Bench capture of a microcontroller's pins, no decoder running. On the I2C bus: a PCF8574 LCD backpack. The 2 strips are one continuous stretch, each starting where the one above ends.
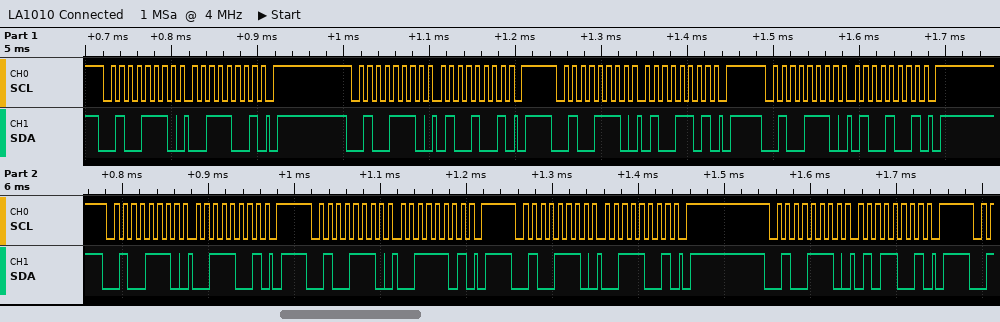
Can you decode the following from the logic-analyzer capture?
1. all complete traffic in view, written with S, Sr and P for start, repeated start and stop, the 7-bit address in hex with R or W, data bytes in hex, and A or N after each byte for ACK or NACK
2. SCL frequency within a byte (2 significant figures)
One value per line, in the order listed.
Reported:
S 27W A 39 A P S 27W A 49 A P S 27W A 4D A P S 27W A 49 A P S 27W A 39 A P S 27W A 3D A P S 27W A 39 A P S 27W A 59 A P
100 kHz
